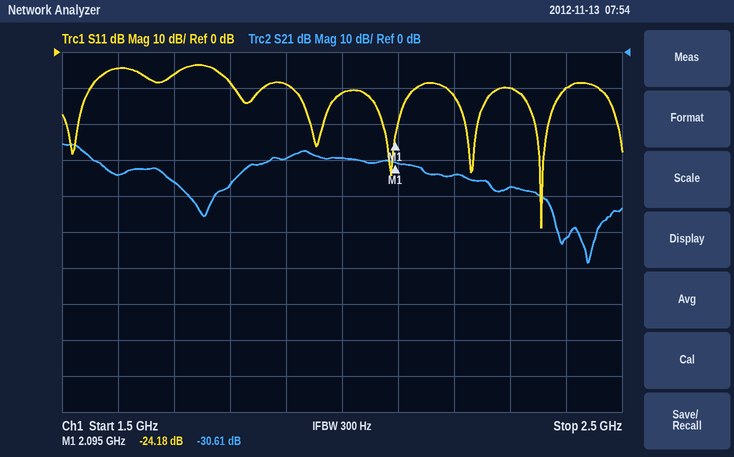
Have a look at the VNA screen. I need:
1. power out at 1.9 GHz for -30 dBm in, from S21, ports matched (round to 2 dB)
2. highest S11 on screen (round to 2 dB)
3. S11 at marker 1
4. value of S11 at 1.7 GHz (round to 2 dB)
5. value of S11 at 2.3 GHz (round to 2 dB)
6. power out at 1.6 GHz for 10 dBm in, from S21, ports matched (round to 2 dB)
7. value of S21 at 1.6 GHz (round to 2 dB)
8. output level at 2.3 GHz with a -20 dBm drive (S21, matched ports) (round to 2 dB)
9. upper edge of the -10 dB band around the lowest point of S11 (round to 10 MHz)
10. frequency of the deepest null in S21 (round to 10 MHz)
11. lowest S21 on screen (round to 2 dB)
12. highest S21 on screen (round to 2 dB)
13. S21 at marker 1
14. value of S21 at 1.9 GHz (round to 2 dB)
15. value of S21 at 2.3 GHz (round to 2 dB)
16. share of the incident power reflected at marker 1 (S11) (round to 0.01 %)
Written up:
-60 dBm
-4 dB
-24.18 dB
-6 dB
-10 dB
-24 dBm
-34 dB
-58 dBm
2.40 GHz
2.44 GHz
-58 dB
-26 dB
-30.61 dB
-30 dB
-38 dB
0.38 %
